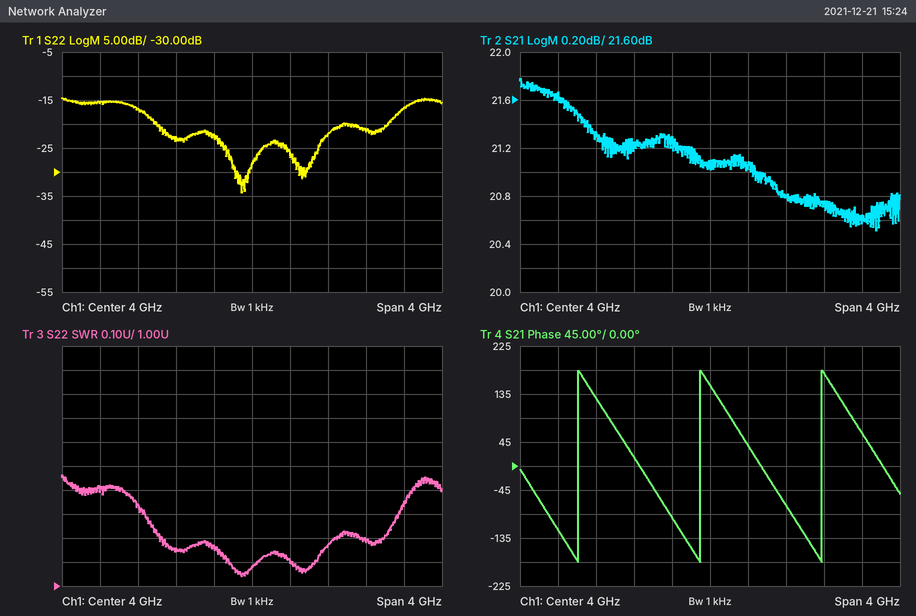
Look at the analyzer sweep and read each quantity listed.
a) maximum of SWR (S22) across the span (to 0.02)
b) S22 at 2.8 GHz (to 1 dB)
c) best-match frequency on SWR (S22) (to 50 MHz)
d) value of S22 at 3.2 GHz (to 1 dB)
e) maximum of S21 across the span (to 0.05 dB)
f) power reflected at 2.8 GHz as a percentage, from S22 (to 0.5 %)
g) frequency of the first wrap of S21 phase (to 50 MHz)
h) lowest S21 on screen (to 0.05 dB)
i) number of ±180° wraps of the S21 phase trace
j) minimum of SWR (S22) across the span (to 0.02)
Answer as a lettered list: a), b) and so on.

a) 1.46
b) -17 dB
c) 3.90 GHz
d) -23 dB
e) 21.80 dB
f) 2.0 %
g) 2.60 GHz
h) 20.50 dB
i) 3
j) 1.04
